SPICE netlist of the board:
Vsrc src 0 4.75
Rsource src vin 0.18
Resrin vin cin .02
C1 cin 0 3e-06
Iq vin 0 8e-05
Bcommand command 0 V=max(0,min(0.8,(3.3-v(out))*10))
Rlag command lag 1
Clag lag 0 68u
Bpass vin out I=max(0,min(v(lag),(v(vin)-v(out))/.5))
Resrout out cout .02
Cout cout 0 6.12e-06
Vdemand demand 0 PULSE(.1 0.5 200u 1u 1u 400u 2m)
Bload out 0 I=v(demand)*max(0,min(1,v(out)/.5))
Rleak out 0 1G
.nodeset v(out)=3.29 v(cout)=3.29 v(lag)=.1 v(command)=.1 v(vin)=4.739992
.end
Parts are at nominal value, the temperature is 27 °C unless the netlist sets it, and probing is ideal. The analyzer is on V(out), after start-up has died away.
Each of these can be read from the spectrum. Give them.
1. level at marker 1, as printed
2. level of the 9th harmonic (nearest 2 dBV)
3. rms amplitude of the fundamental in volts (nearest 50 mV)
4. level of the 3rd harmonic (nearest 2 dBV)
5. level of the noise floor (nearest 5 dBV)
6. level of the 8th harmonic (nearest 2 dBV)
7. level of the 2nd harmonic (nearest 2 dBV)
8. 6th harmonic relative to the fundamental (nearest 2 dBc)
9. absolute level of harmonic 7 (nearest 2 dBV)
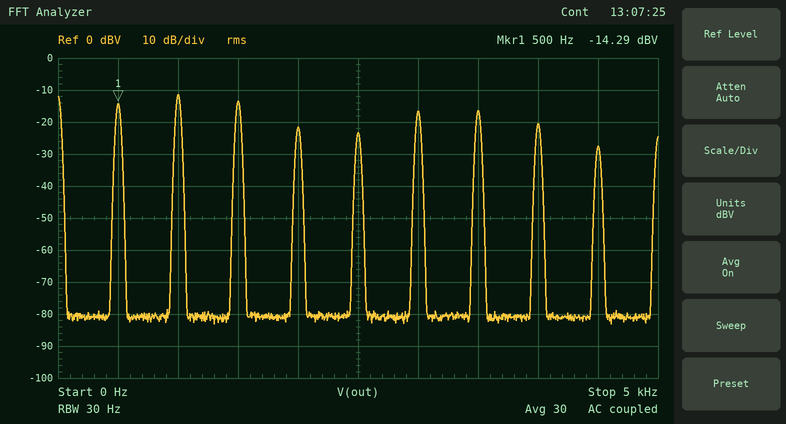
-14.29 dBV
-28 dBV
200 mV
-14 dBV
-80 dBV
-20 dBV
-12 dBV
-2 dBc
-16 dBV
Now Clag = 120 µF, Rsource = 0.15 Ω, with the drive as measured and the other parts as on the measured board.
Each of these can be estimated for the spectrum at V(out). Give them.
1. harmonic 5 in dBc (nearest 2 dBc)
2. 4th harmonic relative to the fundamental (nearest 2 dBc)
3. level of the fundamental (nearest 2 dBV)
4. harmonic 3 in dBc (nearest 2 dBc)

-8 dBc
-10 dBc
-8 dBV
-2 dBc
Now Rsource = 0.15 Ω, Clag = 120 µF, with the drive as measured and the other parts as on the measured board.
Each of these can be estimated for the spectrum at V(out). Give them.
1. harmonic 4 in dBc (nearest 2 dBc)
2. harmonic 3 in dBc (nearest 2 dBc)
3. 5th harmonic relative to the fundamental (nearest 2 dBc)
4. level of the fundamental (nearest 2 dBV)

-10 dBc
-2 dBc
-8 dBc
-8 dBV
